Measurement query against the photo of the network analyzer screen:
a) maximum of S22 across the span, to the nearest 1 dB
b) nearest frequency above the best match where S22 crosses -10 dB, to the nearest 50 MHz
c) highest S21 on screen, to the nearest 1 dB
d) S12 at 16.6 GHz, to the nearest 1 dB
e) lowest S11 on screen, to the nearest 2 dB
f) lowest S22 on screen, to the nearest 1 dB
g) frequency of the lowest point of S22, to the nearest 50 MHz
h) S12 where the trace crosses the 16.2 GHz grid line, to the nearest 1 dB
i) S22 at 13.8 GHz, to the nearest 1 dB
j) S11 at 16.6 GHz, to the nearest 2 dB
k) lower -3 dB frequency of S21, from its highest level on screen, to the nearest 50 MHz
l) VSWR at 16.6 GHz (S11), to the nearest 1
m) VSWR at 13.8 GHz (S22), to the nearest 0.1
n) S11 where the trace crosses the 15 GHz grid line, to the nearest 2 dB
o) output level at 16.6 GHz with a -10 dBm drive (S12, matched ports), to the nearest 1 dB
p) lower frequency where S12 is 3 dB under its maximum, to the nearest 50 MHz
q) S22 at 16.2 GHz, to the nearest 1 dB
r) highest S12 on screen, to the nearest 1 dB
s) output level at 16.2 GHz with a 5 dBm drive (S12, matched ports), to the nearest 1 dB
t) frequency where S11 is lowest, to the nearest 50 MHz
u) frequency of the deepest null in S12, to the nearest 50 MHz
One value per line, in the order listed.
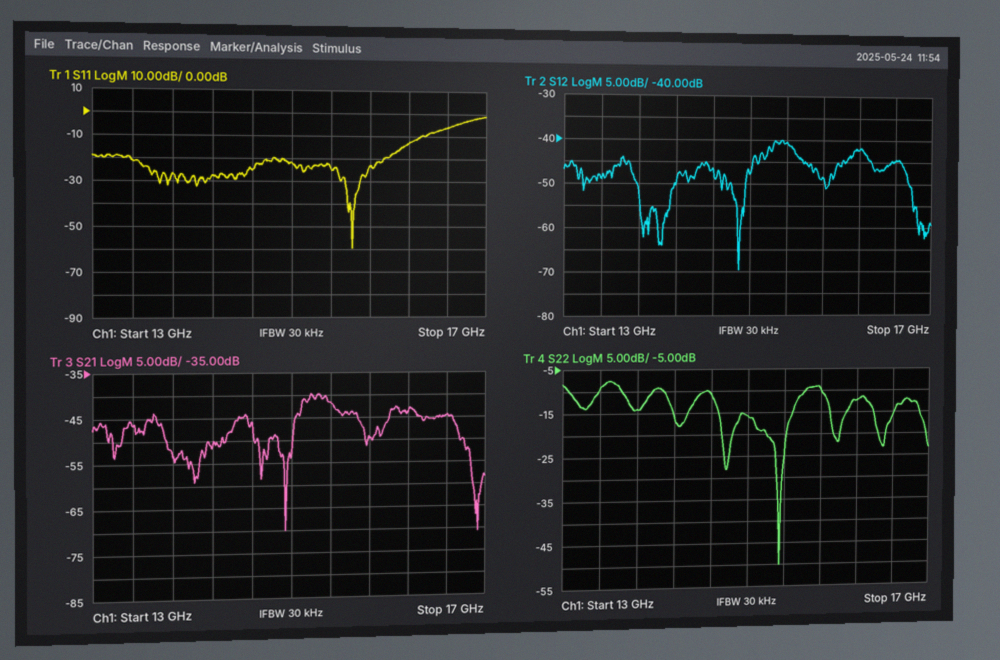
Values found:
-8 dB
15.65 GHz
-40 dB
-45 dB
-60 dB
-50 dB
15.35 GHz
-42 dB
-14 dB
-6 dB
15.10 GHz
3
1.5
-22 dB
-55 dBm
15.20 GHz
-12 dB
-40 dB
-37 dBm
15.60 GHz
14.90 GHz
